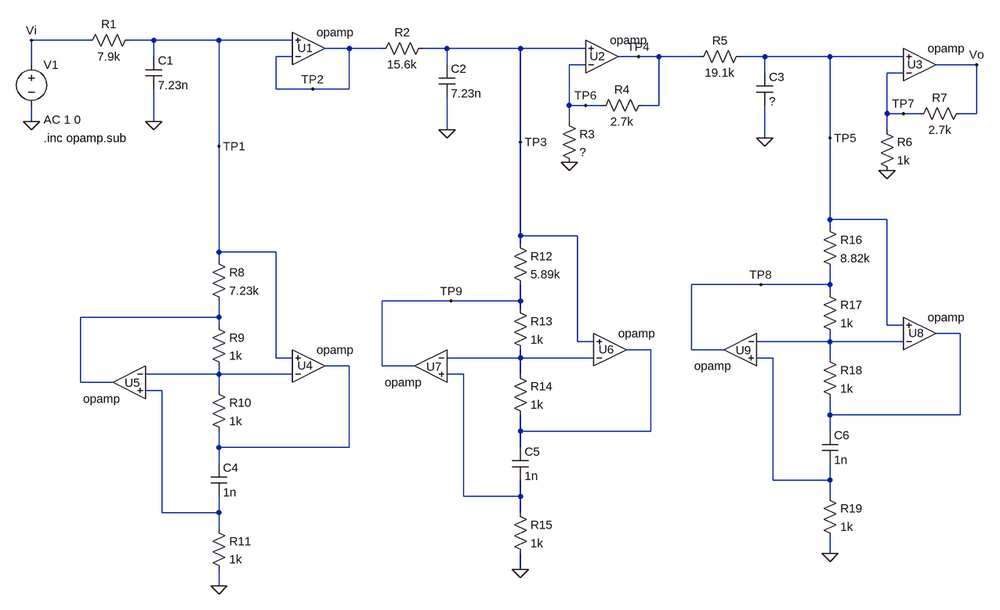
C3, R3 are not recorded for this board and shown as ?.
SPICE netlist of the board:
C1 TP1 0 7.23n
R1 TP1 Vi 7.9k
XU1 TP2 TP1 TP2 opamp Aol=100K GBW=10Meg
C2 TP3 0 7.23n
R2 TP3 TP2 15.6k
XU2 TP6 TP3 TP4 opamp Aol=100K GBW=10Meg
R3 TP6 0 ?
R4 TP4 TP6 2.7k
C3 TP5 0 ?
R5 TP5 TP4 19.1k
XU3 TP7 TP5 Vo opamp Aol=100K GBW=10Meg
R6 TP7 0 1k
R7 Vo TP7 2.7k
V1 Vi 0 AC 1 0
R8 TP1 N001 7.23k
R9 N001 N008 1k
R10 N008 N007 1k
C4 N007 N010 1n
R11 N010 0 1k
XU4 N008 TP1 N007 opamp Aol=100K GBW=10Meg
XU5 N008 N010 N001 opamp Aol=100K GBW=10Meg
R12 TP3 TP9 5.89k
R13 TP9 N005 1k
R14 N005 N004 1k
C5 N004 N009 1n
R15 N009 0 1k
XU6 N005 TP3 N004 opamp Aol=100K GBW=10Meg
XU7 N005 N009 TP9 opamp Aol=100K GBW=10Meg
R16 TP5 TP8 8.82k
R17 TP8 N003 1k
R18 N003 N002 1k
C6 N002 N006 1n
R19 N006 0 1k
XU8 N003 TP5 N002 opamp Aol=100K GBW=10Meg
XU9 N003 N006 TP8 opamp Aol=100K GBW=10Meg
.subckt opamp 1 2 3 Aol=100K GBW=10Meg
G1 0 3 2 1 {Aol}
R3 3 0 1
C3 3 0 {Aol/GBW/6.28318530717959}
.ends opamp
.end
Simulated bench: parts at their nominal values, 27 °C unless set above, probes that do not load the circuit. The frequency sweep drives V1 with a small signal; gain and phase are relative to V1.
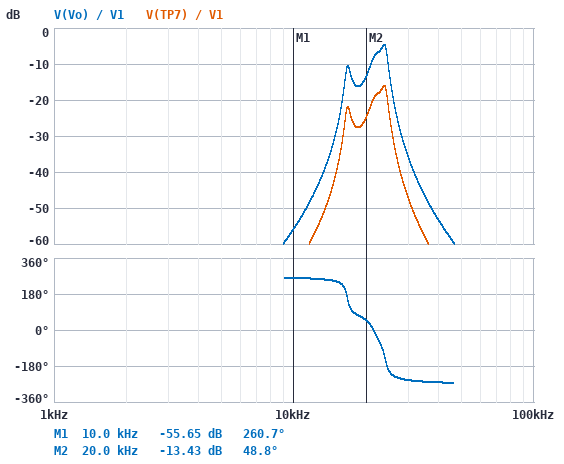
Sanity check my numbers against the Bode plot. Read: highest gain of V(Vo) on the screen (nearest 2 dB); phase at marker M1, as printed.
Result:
-4 dB
260.7 deg
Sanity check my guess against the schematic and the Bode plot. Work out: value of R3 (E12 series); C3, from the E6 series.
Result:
820 Ω
10 nF
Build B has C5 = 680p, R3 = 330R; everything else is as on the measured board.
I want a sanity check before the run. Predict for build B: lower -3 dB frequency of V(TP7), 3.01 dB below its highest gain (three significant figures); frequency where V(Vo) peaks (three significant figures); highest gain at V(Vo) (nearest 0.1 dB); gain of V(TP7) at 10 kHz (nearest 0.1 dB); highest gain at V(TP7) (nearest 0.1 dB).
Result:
16.4 kHz
16.7 kHz
-9.4 dB
-64.2 dB
-20.7 dB
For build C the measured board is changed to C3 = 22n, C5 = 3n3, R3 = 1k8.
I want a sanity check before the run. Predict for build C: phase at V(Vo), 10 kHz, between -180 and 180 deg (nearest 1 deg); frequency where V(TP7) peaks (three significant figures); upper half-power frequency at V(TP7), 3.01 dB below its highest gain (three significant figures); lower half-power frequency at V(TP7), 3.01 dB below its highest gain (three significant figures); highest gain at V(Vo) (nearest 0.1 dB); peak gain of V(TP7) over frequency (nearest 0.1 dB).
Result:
-113 deg
11.3 kHz
11.5 kHz
11.1 kHz
-12.2 dB
-23.6 dB
